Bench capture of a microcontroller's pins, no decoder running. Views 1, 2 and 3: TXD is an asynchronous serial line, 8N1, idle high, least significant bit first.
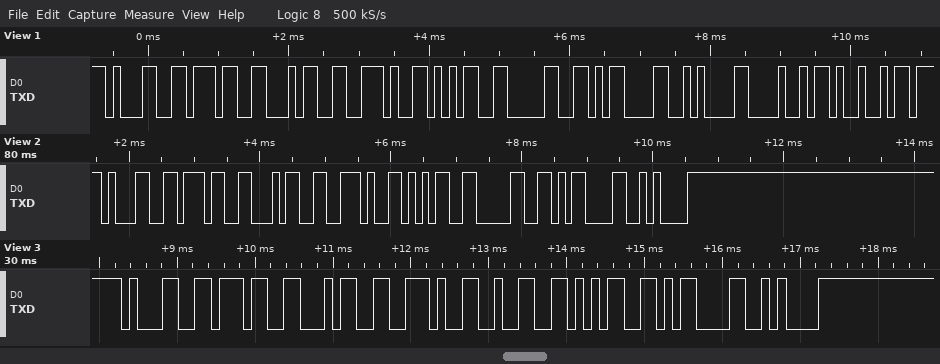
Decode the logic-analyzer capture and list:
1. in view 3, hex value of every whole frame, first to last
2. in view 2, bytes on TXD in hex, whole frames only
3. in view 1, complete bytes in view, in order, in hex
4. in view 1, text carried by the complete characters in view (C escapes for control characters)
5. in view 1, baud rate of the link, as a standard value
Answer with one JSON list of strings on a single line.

["31 37 34 2E 32 35 0D 0A", "31 37 34 2E 35 30 0D 0A", "31 37 34 2E 35 30 0D 0A 48 49", "\"174.50\\r\\nHI\"", "9600 baud"]
